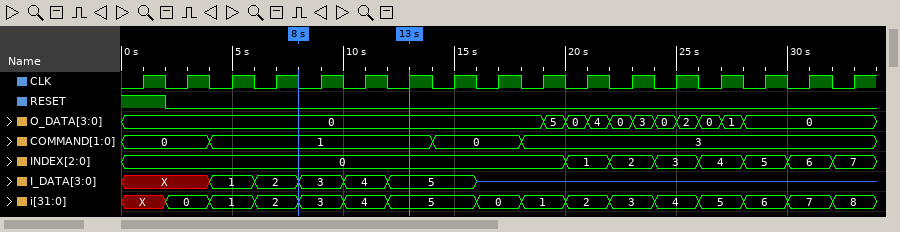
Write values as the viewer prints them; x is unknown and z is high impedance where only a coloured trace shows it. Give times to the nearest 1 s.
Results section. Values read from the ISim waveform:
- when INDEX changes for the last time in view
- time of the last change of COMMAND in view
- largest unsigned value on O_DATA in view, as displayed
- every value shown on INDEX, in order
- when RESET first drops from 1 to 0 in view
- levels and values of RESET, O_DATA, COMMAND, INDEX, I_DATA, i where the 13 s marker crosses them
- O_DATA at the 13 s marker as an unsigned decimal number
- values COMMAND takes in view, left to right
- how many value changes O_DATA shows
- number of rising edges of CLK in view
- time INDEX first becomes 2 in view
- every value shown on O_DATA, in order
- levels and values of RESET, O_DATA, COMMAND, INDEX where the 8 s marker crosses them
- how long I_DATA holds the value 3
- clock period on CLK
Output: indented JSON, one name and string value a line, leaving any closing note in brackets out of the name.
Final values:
{
  "when INDEX changes for the last time in view": "32 s",
  "time of the last change of COMMAND in view": "18 s",
  "largest unsigned value on O_DATA in view, as displayed": "5",
  "every value shown on INDEX, in order": "0, 1, 2, 3, 4, 5, 6, 7",
  "when RESET first drops from 1 to 0 in view": "2 s",
  "levels and values of RESET, O_DATA, COMMAND, INDEX, I_DATA, i where the 13 s marker crosses them": "RESET=0, O_DATA=0, COMMAND=1, INDEX=0, I_DATA=5, i=5",
  "O_DATA at the 13 s marker as an unsigned decimal number": "0",
  "values COMMAND takes in view, left to right": "0, 1, 0, 3",
  "how many value changes O_DATA shows": "10",
  "number of rising edges of CLK in view": "17",
  "time INDEX first becomes 2 in view": "22 s",
  "every value shown on O_DATA, in order": "0, 5, 0, 4, 0, 3, 0, 2, 0, 1, 0",
  "levels and values of RESET, O_DATA, COMMAND, INDEX where the 8 s marker crosses them": "RESET=0, O_DATA=0, COMMAND=1, INDEX=0",
  "how long I_DATA holds the value 3": "2 s",
  "clock period on CLK": "2 s"
}
